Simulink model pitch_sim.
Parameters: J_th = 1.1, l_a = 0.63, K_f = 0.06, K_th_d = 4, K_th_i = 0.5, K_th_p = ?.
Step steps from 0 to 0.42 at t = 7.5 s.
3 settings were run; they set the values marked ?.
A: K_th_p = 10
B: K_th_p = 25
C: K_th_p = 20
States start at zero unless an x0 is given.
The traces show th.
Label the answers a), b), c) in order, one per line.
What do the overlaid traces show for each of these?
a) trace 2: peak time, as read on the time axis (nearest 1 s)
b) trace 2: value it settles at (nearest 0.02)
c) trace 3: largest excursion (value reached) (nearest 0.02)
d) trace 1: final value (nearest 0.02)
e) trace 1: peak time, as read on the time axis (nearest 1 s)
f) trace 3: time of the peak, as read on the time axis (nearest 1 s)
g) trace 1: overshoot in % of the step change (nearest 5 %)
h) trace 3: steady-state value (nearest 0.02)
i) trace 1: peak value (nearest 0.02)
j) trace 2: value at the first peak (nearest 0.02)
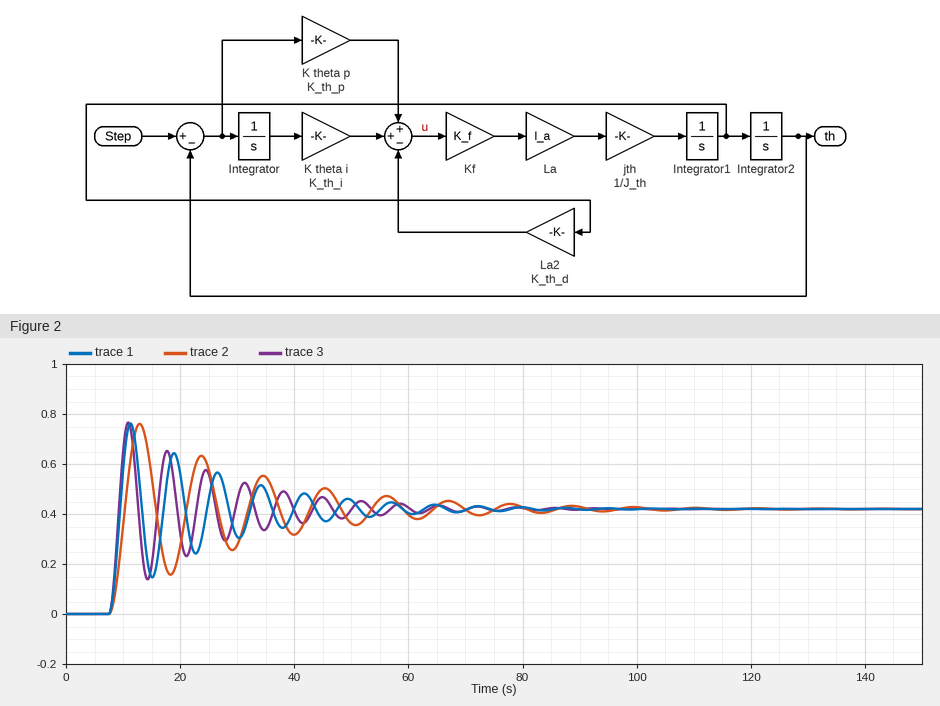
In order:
a) 13 s
b) 0.42
c) 0.76
d) 0.42
e) 11 s
f) 11 s
g) 80 %
h) 0.42
i) 0.76
j) 0.76
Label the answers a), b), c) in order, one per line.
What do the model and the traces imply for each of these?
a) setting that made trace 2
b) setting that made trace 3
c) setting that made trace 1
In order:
a) A
b) B
c) C
